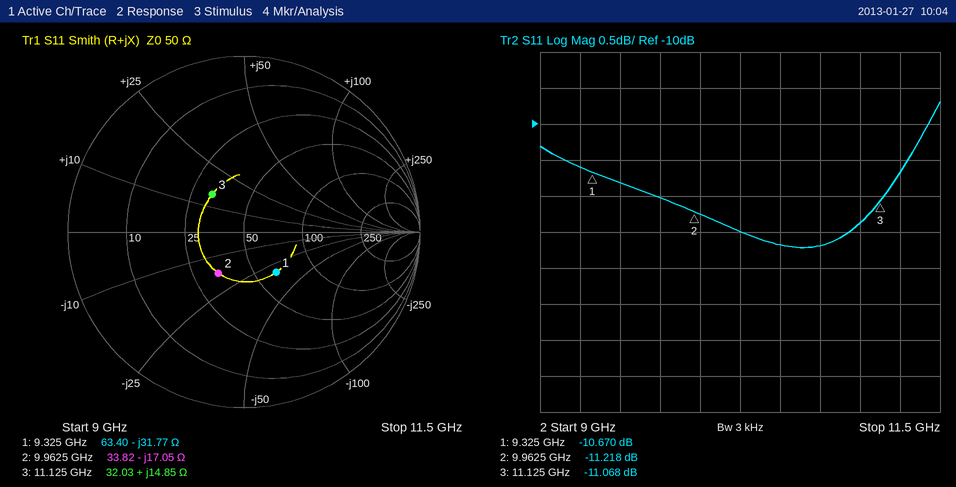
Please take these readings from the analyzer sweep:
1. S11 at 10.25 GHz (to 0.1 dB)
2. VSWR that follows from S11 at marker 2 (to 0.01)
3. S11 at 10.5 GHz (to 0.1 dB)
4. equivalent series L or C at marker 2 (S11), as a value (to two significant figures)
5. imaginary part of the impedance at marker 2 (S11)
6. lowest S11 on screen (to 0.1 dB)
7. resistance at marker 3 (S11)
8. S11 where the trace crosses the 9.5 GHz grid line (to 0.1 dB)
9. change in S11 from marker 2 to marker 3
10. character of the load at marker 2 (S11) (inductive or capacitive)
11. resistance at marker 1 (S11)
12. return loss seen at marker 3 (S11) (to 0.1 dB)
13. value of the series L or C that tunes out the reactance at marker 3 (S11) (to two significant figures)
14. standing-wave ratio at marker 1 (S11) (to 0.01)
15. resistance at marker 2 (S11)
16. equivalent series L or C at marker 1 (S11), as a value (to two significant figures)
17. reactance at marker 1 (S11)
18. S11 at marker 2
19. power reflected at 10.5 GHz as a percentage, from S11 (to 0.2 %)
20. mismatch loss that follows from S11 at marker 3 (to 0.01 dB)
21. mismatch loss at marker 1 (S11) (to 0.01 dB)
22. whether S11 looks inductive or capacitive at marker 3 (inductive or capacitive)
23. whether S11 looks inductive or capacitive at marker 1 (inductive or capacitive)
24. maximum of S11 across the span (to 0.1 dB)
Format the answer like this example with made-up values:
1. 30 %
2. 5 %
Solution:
1. -11.5 dB
2. 1.76
3. -11.7 dB
4. 940 fF
5. -17.05 Ω
6. -11.7 dB
7. 32.03 Ω
8. -10.8 dB
9. 0.150 dB
10. capacitive
11. 63.40 Ω
12. 11.1 dB
13. 960 fF
14. 1.83
15. 33.82 Ω
16. 540 fF
17. -31.77 Ω
18. -11.218 dB
19. 6.8 %
20. 0.35 dB
21. 0.39 dB
22. inductive
23. capacitive
24. -9.7 dB
